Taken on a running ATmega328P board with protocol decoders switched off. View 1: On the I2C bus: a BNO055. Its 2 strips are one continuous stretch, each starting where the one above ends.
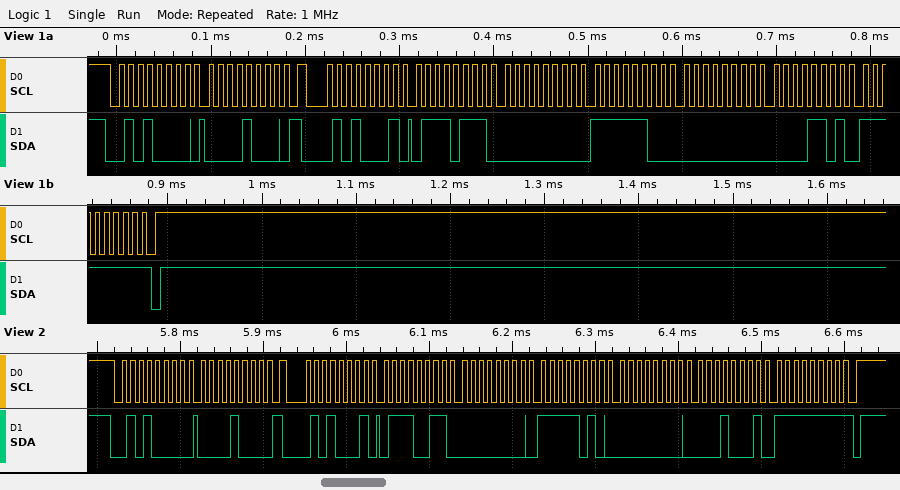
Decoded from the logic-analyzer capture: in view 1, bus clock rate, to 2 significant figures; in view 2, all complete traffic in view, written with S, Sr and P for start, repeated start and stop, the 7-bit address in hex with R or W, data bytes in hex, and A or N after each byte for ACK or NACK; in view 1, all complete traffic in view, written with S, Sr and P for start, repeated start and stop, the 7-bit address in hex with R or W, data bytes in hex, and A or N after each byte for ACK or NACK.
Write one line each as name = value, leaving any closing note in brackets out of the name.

in view 1, bus clock rate, to 2 significant figures = 100 kHz
in view 2, all complete traffic in view, written with S, Sr and P for start, repeated start and stop, the 7-bit address in hex with R or W, data bytes in hex, and A or N after each byte for ACK or NACK = S 28W A 08 A Sr 28R A 73 A 00 A FA A 00 A 11 A FF N P
in view 1, all complete traffic in view, written with S, Sr and P for start, repeated start and stop, the 7-bit address in hex with R or W, data bytes in hex, and A or N after each byte for ACK or NACK = S 28W A 08 A Sr 28R A 77 A 00 A FC A 00 A 0D A FF N P
